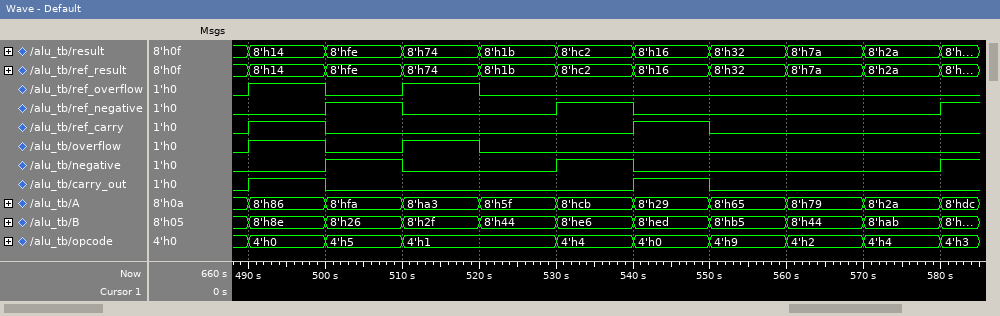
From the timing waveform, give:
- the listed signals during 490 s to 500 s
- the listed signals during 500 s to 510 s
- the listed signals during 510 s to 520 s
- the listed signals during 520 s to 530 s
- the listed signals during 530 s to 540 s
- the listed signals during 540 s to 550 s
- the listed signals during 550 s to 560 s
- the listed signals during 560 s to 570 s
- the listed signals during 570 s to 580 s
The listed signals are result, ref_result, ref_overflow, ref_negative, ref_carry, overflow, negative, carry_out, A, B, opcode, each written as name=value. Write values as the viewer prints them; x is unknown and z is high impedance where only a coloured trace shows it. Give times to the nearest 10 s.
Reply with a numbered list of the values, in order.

1. result=8'h14, ref_result=8'h14, ref_overflow=1, ref_negative=0, ref_carry=1, overflow=1, negative=0, carry_out=1, A=8'h86, B=8'h8e, opcode=4'h0
2. result=8'hfe, ref_result=8'hfe, ref_overflow=0, ref_negative=1, ref_carry=0, overflow=0, negative=1, carry_out=0, A=8'hfa, B=8'h26, opcode=4'h5
3. result=8'h74, ref_result=8'h74, ref_overflow=1, ref_negative=0, ref_carry=0, overflow=1, negative=0, carry_out=0, A=8'ha3, B=8'h2f, opcode=4'h1
4. result=8'h1b, ref_result=8'h1b, ref_overflow=0, ref_negative=0, ref_carry=0, overflow=0, negative=0, carry_out=0, A=8'h5f, B=8'h44, opcode=4'h1
5. result=8'hc2, ref_result=8'hc2, ref_overflow=0, ref_negative=1, ref_carry=0, overflow=0, negative=1, carry_out=0, A=8'hcb, B=8'he6, opcode=4'h4
6. result=8'h16, ref_result=8'h16, ref_overflow=0, ref_negative=0, ref_carry=1, overflow=0, negative=0, carry_out=1, A=8'h29, B=8'hed, opcode=4'h0
7. result=8'h32, ref_result=8'h32, ref_overflow=0, ref_negative=0, ref_carry=0, overflow=0, negative=0, carry_out=0, A=8'h65, B=8'hb5, opcode=4'h9
8. result=8'h7a, ref_result=8'h7a, ref_overflow=0, ref_negative=0, ref_carry=0, overflow=0, negative=0, carry_out=0, A=8'h79, B=8'h44, opcode=4'h2
9. result=8'h2a, ref_result=8'h2a, ref_overflow=0, ref_negative=0, ref_carry=0, overflow=0, negative=0, carry_out=0, A=8'h2a, B=8'hab, opcode=4'h4
